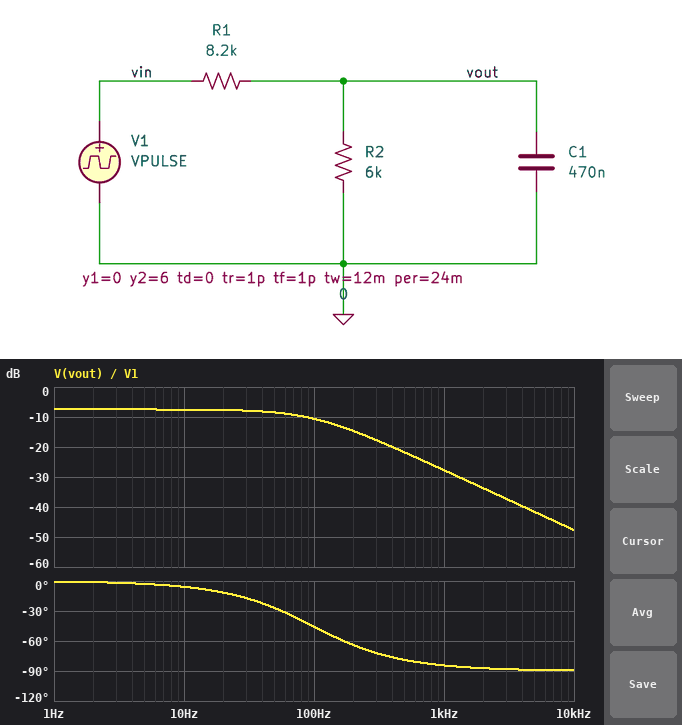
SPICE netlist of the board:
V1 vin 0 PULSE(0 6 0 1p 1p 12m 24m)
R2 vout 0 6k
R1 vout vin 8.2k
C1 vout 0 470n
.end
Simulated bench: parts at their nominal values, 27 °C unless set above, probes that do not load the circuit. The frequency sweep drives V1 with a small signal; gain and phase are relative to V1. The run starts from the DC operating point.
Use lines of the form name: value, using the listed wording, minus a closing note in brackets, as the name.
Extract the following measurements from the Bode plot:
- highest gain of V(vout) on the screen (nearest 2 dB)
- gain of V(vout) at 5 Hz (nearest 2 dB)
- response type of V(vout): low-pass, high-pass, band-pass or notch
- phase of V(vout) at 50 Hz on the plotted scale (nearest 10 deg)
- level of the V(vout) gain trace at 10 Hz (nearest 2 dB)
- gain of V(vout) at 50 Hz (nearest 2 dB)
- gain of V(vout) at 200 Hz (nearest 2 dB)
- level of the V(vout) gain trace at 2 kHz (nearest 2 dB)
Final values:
highest gain of V(vout) on the screen: -8 dB
gain of V(vout) at 5 Hz: -8 dB
response type of V(vout): low-pass, high-pass, band-pass or notch: low-pass
phase of V(vout) at 50 Hz on the plotted scale: -30 deg
level of the V(vout) gain trace at 10 Hz: -8 dB
gain of V(vout) at 50 Hz: -8 dB
gain of V(vout) at 200 Hz: -14 dB
level of the V(vout) gain trace at 2 kHz: -34 dB
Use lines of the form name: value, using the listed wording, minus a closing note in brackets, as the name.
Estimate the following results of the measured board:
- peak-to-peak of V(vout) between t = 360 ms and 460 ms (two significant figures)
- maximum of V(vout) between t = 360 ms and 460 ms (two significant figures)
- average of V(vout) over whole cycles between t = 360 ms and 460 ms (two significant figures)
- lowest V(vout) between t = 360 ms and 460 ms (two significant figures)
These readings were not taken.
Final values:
peak-to-peak of V(vout) between t = 360 ms and 460 ms: 2.5 V
maximum of V(vout) between t = 360 ms and 460 ms: 2.5 V
average of V(vout) over whole cycles between t = 360 ms and 460 ms: 1.3 V
lowest V(vout) between t = 360 ms and 460 ms: 1.6 mV
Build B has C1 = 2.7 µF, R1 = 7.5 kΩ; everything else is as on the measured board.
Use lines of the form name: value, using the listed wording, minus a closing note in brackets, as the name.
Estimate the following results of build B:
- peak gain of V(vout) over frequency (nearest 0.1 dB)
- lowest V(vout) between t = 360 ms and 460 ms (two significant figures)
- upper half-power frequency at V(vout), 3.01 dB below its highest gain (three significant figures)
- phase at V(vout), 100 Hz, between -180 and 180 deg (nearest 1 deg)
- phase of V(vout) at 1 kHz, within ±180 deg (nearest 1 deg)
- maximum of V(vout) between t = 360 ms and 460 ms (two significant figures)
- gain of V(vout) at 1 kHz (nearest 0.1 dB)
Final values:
peak gain of V(vout) over frequency: -7.0 dB
lowest V(vout) between t = 360 ms and 460 ms: 560 mV
upper half-power frequency at V(vout), 3.01 dB below its highest gain: 17.7 Hz
phase at V(vout), 100 Hz, between -180 and 180 deg: -80 deg
phase of V(vout) at 1 kHz, within ±180 deg: -89 deg
maximum of V(vout) between t = 360 ms and 460 ms: 2.1 V
gain of V(vout) at 1 kHz: -42.1 dB
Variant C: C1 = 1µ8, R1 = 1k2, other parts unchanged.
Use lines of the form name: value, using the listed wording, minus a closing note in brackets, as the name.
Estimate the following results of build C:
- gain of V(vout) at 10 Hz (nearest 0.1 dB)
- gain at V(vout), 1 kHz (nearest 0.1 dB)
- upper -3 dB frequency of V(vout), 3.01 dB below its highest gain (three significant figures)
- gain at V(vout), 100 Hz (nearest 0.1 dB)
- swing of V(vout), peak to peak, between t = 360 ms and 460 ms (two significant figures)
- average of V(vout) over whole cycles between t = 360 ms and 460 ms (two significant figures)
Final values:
gain of V(vout) at 10 Hz: -1.6 dB
gain at V(vout), 1 kHz: -22.7 dB
upper -3 dB frequency of V(vout), 3.01 dB below its highest gain: 88.4 Hz
gain at V(vout), 100 Hz: -5.2 dB
swing of V(vout), peak to peak, between t = 360 ms and 460 ms: 5.0 V
average of V(vout) over whole cycles between t = 360 ms and 460 ms: 2.5 V
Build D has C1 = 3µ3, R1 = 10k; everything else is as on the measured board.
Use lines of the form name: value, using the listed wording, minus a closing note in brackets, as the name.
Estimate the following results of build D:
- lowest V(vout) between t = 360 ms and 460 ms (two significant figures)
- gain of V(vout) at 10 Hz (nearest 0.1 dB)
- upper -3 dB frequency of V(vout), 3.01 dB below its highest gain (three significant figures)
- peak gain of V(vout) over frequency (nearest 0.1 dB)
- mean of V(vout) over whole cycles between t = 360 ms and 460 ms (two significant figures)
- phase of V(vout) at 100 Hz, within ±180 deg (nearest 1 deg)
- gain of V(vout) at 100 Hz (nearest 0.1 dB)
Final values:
lowest V(vout) between t = 360 ms and 460 ms: 620 mV
gain of V(vout) at 10 Hz: -10.6 dB
upper -3 dB frequency of V(vout), 3.01 dB below its highest gain: 12.9 Hz
peak gain of V(vout) over frequency: -8.5 dB
mean of V(vout) over whole cycles between t = 360 ms and 460 ms: 1.1 V
phase of V(vout) at 100 Hz, within ±180 deg: -83 deg
gain of V(vout) at 100 Hz: -26.4 dB
